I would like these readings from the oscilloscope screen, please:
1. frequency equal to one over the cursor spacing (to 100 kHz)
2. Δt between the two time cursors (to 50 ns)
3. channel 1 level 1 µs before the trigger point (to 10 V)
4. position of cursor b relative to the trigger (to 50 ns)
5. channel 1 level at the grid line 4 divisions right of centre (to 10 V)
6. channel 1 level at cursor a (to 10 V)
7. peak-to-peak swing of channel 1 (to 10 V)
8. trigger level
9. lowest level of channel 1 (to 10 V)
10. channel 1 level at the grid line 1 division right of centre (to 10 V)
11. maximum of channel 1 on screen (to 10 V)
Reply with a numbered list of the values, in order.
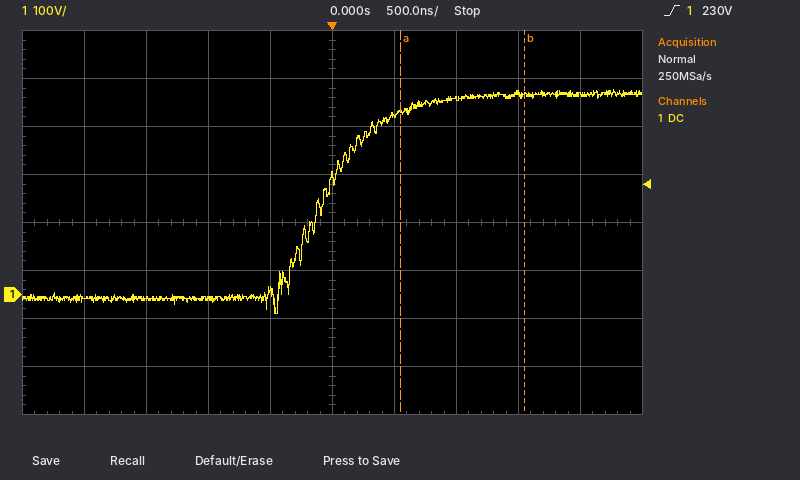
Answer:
1. 1.0 MHz
2. 1.00 µs
3. -10 V
4. +1.55 µs
5. 420 V
6. 380 V
7. 470 V
8. 230 V
9. -40 V
10. 370 V
11. 430 V
